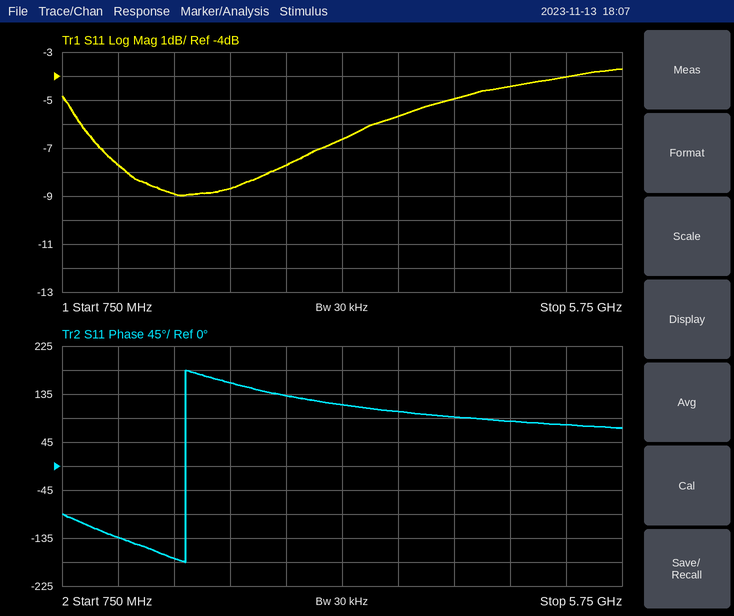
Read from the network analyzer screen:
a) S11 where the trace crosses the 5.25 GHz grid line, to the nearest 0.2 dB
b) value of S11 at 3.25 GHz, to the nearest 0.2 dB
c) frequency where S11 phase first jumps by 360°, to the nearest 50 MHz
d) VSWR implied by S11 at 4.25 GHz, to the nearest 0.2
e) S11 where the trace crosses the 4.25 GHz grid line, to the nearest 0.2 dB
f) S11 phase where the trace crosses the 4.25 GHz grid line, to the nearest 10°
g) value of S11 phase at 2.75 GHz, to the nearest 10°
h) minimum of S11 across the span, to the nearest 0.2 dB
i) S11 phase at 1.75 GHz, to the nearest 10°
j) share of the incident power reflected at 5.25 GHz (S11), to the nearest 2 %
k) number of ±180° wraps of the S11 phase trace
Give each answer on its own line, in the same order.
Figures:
-4.0 dB
-6.6 dB
1.85 GHz
3.6
-5.0 dB
90°
130°
-9.0 dB
-170°
40 %
1
